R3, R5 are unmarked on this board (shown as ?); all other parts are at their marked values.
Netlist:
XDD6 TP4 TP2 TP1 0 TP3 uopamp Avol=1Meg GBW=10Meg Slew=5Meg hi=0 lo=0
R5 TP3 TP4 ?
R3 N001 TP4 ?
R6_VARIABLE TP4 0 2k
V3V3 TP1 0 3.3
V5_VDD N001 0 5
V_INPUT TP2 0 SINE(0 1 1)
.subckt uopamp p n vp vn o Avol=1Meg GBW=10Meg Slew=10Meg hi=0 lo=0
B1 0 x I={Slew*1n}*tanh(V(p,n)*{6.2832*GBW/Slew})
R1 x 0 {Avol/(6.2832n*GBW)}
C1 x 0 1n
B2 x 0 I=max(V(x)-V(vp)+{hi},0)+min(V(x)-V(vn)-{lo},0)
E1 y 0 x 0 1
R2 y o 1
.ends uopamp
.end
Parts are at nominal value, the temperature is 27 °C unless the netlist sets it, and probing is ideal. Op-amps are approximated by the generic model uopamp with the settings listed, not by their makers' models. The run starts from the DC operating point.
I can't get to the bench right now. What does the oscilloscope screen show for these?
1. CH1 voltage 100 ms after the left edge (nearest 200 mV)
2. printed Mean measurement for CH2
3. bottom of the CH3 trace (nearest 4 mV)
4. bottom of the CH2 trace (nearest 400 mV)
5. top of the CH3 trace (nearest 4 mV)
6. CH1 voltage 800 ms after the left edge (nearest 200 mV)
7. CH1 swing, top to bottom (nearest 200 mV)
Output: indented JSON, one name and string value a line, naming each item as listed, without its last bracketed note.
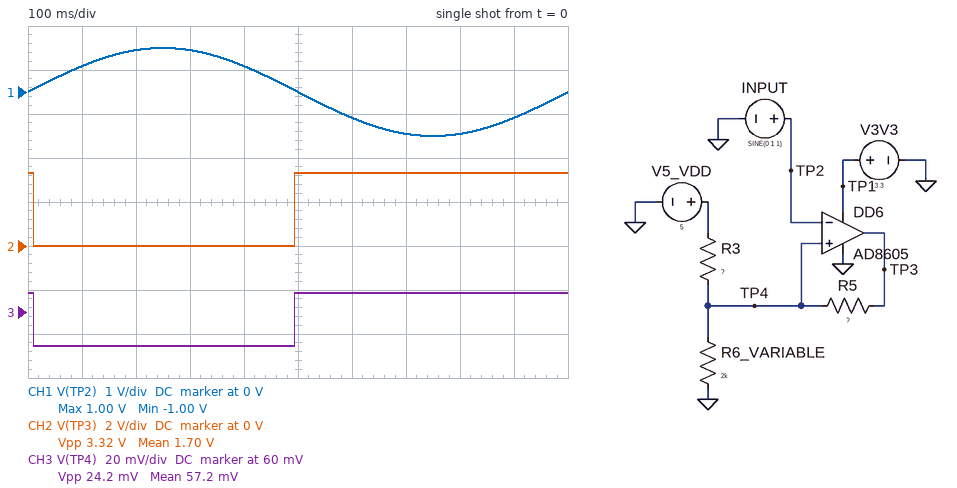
{
  "CH1 voltage 100 ms after the left edge": "600 mV",
  "printed Mean measurement for CH2": "1.70 V",
  "bottom of the CH3 trace": "44 mV",
  "bottom of the CH2 trace": "0 V",
  "top of the CH3 trace": "68 mV",
  "CH1 voltage 800 ms after the left edge": "-1.0 V",
  "CH1 swing, top to bottom": "2.0 V"
}
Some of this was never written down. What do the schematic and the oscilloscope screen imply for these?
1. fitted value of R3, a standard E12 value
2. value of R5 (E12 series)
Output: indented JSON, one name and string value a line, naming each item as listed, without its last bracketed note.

{
  "fitted value of R3, a standard E12 value": "220 kΩ",
  "value of R5": "270 kΩ"
}
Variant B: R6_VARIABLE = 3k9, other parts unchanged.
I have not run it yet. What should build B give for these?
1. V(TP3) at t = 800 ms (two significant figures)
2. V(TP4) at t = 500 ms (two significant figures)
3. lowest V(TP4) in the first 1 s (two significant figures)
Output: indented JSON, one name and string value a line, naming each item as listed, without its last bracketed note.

{
  "V(TP3) at t = 800 ms": "3.3 V",
  "V(TP4) at t = 500 ms": "130 mV",
  "lowest V(TP4) in the first 1 s": "86 mV"
}
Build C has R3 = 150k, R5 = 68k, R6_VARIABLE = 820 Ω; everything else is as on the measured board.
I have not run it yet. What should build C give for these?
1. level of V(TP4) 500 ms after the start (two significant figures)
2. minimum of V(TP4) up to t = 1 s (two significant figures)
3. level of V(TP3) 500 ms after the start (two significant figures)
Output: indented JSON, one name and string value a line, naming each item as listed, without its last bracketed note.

{
  "level of V(TP4) 500 ms after the start": "66 mV",
  "minimum of V(TP4) up to t = 1 s": "27 mV",
  "level of V(TP3) 500 ms after the start": "3.3 V"
}
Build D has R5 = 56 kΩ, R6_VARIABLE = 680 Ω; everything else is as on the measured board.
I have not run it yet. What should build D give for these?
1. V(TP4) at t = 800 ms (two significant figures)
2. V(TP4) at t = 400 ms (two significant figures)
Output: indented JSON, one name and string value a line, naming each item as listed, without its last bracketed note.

{
  "V(TP4) at t = 800 ms": "55 mV",
  "V(TP4) at t = 400 ms": "15 mV"
}
